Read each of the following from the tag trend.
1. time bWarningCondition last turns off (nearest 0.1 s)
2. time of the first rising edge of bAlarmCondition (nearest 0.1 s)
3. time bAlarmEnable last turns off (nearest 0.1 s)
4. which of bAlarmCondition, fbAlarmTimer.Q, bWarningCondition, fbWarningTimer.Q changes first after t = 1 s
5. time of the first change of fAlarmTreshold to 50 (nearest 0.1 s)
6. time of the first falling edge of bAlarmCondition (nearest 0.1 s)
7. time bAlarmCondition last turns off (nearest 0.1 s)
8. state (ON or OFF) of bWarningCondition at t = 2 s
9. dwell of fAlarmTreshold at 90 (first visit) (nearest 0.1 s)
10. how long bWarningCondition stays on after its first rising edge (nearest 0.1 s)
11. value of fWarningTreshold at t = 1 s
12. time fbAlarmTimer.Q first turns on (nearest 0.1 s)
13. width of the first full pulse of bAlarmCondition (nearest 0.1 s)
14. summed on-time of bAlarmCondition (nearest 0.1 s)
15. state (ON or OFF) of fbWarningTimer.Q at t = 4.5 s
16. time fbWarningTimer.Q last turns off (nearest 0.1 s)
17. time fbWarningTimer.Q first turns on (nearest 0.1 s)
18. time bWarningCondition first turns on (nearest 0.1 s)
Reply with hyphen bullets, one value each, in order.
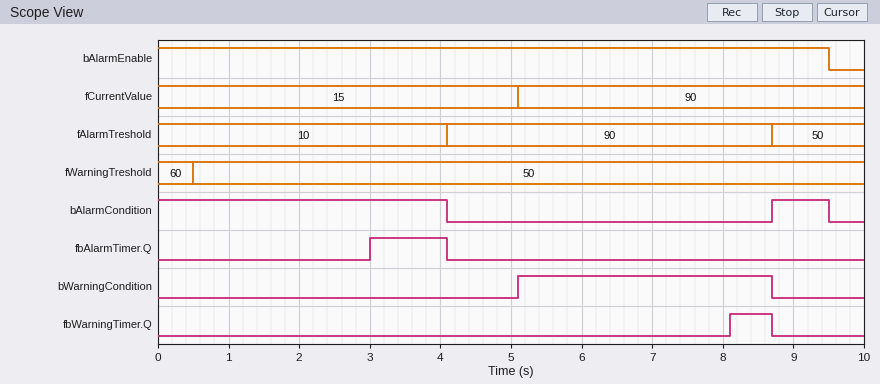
- 8.7 s
- 8.7 s
- 9.5 s
- fbAlarmTimer.Q
- 8.7 s
- 4.1 s
- 9.5 s
- OFF
- 4.6 s
- 3.6 s
- 50
- 3.0 s
- 0.8 s
- 4.9 s
- OFF
- 8.7 s
- 8.1 s
- 5.1 s
